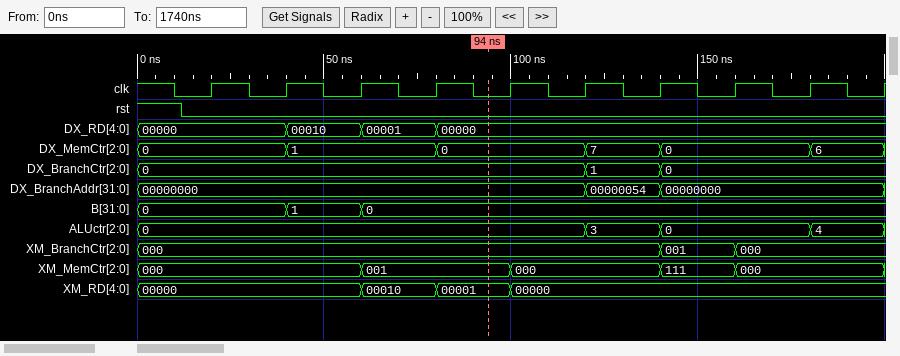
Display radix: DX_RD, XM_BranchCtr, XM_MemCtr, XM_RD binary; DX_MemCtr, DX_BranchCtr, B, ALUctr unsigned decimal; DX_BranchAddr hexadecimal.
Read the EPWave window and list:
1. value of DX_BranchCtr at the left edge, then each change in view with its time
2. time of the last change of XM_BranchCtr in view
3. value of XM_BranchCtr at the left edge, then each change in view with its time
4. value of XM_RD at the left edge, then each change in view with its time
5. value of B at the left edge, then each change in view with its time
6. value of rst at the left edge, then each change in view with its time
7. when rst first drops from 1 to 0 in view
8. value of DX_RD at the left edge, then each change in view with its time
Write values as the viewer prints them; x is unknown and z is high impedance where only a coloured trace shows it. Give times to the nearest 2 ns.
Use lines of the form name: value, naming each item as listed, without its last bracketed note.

value of DX_BranchCtr at the left edge, then each change in view with its time: 0, 1 at 120 ns, 0 at 140 ns
time of the last change of XM_BranchCtr in view: 160 ns
value of XM_BranchCtr at the left edge, then each change in view with its time: 000, 001 at 140 ns, 000 at 160 ns
value of XM_RD at the left edge, then each change in view with its time: 00000, 00010 at 60 ns, 00001 at 80 ns, 00000 at 100 ns
value of B at the left edge, then each change in view with its time: 0, 1 at 40 ns, 0 at 60 ns
value of rst at the left edge, then each change in view with its time: 1, 0 at 12 ns
when rst first drops from 1 to 0 in view: 12 ns
value of DX_RD at the left edge, then each change in view with its time: 00000, 00010 at 40 ns, 00001 at 60 ns, 00000 at 80 ns
